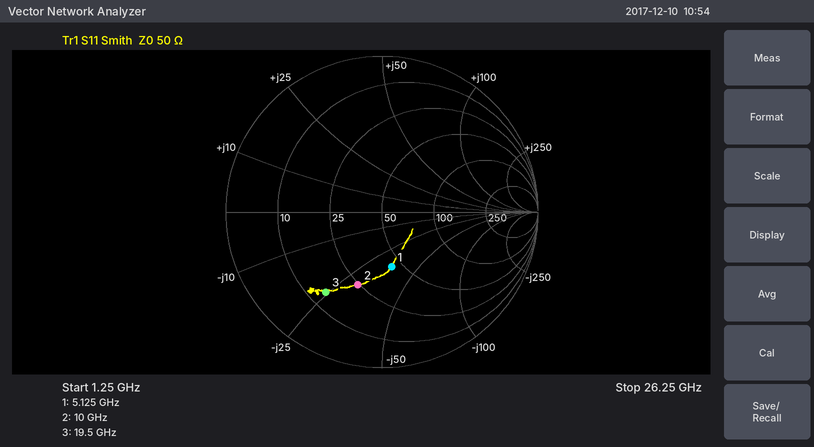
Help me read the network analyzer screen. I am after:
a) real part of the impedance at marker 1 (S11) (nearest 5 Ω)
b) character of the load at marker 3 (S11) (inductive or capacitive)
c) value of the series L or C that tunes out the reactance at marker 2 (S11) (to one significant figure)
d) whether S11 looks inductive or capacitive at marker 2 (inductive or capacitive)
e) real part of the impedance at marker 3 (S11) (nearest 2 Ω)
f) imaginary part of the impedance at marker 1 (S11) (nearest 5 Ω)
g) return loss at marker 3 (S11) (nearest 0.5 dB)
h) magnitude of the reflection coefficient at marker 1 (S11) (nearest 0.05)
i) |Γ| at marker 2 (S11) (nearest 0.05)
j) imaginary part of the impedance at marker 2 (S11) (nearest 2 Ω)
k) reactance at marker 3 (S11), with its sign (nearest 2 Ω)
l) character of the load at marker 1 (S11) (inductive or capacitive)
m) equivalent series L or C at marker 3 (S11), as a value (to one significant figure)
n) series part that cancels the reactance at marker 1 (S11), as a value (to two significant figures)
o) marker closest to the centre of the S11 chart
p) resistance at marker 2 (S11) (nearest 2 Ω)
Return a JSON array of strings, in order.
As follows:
["45 Ω", "capacitive", "500 pH", "capacitive", "14 Ω", "-35 Ω", "4.0 dB", "0.35", "0.50", "-30 Ω", "-24 Ω", "capacitive", "300 fF", "1.1 nH", "marker 1", "24 Ω"]
